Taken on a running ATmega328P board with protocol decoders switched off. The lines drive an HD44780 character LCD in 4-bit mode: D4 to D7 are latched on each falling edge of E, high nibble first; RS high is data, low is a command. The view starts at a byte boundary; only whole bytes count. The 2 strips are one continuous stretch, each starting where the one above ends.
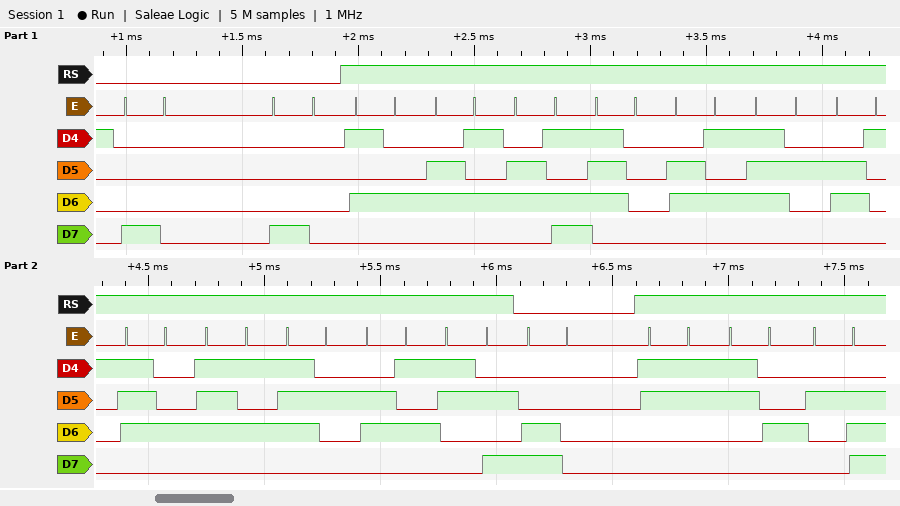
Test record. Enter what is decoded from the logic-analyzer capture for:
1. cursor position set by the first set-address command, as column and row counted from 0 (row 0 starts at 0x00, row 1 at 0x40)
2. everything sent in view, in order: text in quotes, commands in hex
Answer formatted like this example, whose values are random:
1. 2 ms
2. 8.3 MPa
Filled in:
1. column 0, row 0
2. 0x80 0x80 "Temperature:" 0xC0 "34."
